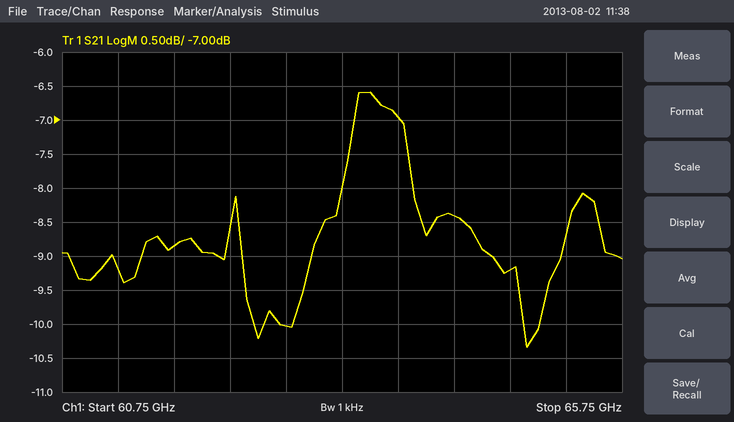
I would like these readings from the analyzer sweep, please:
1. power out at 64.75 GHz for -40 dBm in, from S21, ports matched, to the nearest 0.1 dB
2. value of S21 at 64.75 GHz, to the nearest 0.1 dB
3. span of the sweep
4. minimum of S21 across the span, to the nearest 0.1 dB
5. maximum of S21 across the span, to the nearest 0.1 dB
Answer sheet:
-49.2 dBm
-9.2 dB
5 GHz
-10.3 dB
-6.6 dB
